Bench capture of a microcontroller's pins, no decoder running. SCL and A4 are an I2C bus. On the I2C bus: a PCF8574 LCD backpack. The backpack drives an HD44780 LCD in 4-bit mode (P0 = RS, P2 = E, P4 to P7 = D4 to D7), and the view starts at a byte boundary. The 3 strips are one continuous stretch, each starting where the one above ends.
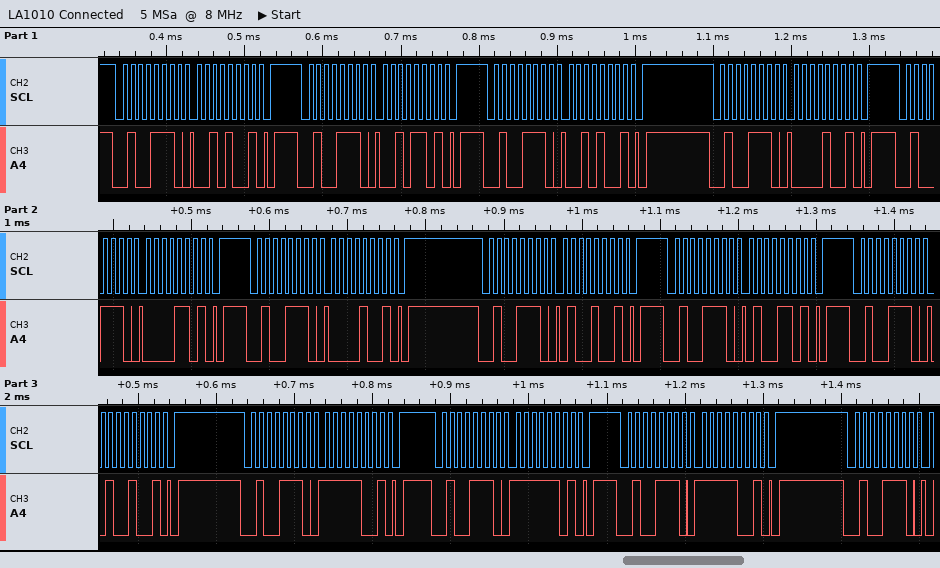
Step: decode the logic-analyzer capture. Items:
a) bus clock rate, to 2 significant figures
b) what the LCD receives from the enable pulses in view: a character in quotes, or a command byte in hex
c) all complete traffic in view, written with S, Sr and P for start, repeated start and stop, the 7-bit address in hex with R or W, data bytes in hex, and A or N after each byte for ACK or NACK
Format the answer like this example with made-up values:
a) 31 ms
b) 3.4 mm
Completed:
a) 100 kHz
b) ' ' 'O'
c) S 27W A 29 A P S 27W A 2D A P S 27W A 29 A P S 27W A 09 A P S 27W A 0D A P S 27W A 09 A P S 27W A 49 A P S 27W A 4D A P S 27W A 49 A P S 27W A F9 A P S 27W A FD A P S 27W A F9 A P S 27W A
